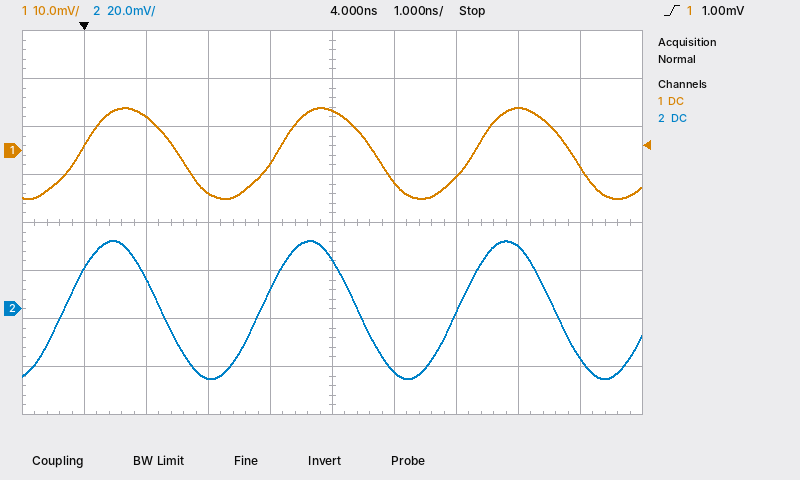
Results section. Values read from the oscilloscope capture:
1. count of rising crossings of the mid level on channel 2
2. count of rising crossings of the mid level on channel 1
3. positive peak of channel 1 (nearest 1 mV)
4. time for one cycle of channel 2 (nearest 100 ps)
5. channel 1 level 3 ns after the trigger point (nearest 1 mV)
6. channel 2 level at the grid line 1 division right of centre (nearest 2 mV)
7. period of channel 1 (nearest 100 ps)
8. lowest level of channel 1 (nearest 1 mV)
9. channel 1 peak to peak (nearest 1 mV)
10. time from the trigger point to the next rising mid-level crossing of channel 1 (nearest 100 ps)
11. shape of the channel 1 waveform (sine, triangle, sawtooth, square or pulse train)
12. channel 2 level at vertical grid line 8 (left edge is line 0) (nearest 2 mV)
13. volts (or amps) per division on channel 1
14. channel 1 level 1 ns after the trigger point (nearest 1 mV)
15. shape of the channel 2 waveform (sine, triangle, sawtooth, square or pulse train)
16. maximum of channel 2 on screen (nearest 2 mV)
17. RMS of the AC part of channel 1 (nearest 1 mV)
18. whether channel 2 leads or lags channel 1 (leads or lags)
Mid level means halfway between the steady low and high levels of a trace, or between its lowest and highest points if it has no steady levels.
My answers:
3
3
9 mV
3.2 ns
-3 mV
-26 mV
3.2 ns
-10 mV
19 mV
3.1 ns
sine
26 mV
10 mV
7 mV
sine
28 mV
7 mV
leads
